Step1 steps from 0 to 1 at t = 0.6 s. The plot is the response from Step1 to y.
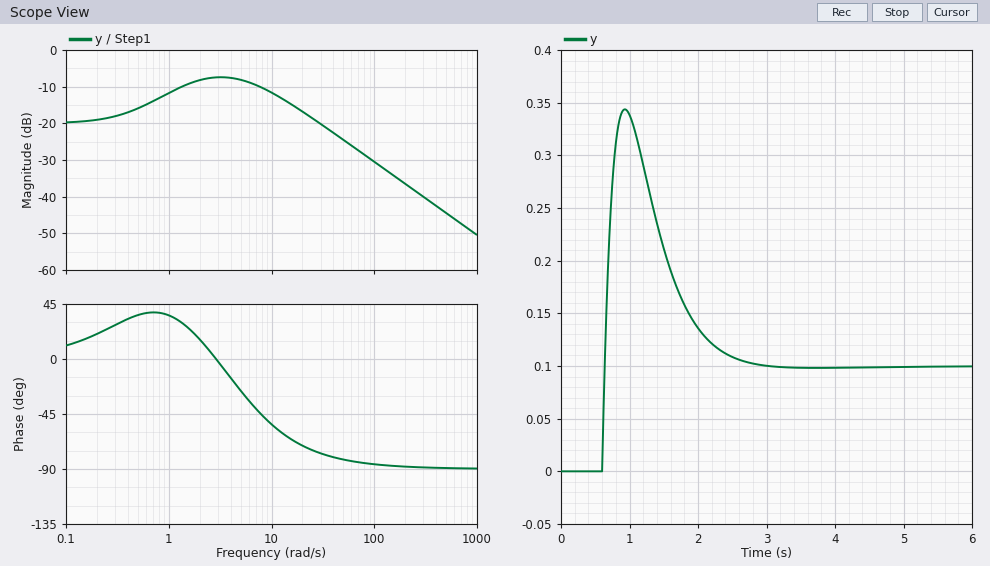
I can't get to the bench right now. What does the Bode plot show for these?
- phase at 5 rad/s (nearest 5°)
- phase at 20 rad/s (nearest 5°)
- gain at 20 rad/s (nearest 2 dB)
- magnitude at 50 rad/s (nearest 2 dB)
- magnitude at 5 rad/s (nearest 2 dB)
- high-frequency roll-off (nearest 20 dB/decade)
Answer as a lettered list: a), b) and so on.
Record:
a) -25°
b) -70°
c) -16 dB
d) -24 dB
e) -8 dB
f) -20 dB/decade
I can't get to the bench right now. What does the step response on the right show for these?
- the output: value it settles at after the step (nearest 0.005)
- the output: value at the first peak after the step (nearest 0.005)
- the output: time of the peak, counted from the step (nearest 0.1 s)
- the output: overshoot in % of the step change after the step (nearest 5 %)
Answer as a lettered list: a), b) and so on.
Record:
a) 0.100
b) 0.345
c) 0.3 s
d) 245 %
